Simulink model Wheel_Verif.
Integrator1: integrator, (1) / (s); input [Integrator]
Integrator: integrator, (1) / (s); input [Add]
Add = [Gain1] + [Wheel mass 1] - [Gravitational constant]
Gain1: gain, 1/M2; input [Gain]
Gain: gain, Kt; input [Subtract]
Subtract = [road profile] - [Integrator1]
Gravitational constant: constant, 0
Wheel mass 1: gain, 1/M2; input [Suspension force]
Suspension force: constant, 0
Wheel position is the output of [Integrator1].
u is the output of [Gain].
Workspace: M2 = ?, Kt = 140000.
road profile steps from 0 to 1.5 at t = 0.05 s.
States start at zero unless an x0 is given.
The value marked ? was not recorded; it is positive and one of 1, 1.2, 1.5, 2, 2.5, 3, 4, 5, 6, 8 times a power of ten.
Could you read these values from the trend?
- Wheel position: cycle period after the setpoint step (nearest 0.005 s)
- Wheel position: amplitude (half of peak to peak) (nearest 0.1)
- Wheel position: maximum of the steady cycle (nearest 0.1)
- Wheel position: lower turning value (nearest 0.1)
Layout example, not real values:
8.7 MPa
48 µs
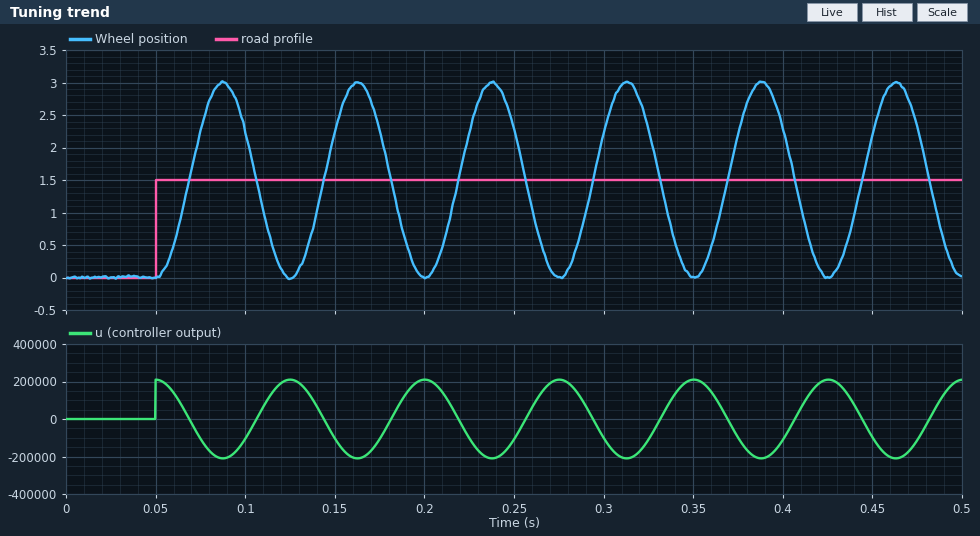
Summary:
0.075 s
1.5
3.0
0.0
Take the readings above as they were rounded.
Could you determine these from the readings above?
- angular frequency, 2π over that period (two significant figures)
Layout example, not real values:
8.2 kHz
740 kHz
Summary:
84 rad/s
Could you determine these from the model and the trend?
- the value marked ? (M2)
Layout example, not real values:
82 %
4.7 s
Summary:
20
